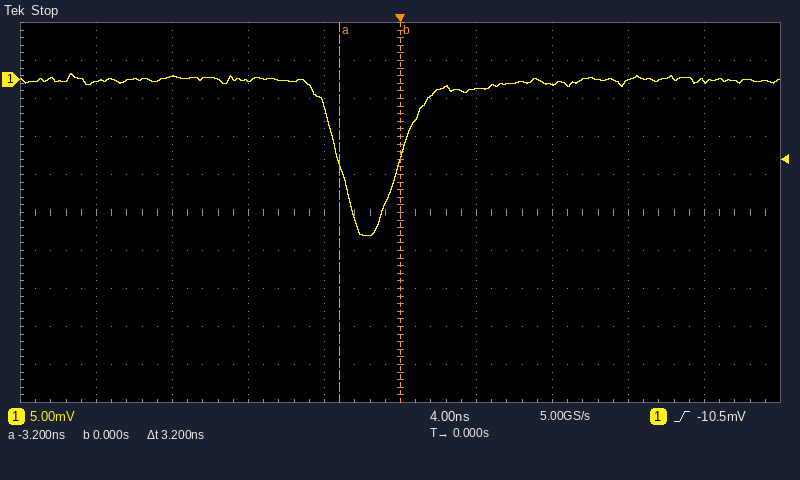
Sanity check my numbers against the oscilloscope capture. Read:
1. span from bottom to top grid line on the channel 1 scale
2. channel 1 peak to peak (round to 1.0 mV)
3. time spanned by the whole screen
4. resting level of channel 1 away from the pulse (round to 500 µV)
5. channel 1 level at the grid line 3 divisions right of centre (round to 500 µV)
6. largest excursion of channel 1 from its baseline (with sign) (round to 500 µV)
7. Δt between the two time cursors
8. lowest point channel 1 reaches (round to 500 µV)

50 mV
21.0 mV
40 ns
0.0 mV
0.0 mV
-20.5 mV
3.2 ns
-20.5 mV
